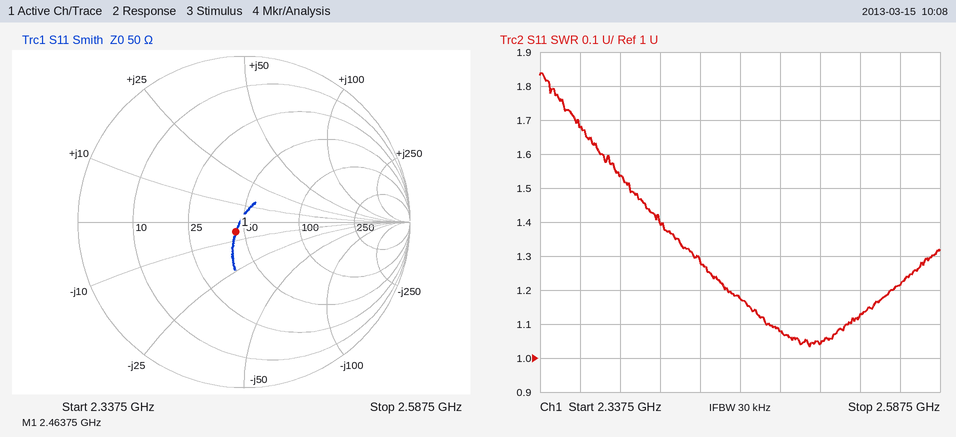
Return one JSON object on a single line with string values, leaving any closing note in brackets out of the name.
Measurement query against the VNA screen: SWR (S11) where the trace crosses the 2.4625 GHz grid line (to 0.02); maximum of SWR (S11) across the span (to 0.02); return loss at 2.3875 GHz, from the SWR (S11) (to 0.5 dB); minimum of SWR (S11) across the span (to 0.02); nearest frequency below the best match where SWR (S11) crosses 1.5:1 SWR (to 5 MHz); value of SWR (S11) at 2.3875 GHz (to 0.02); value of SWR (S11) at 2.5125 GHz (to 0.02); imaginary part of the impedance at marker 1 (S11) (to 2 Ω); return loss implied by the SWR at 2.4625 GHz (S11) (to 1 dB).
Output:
{"SWR (S11) where the trace crosses the 2.4625 GHz grid line": "1.18", "maximum of SWR (S11) across the span": "1.84", "return loss at 2.3875 GHz, from the SWR (S11)": "13.5 dB", "minimum of SWR (S11) across the span": "1.04", "nearest frequency below the best match where SWR (S11) crosses 1.5:1 SWR": "2.395 GHz", "value of SWR (S11) at 2.3875 GHz": "1.54", "value of SWR (S11) at 2.5125 GHz": "1.04", "imaginary part of the impedance at marker 1 (S11)": "-6 Ω", "return loss implied by the SWR at 2.4625 GHz (S11)": "22 dB"}
